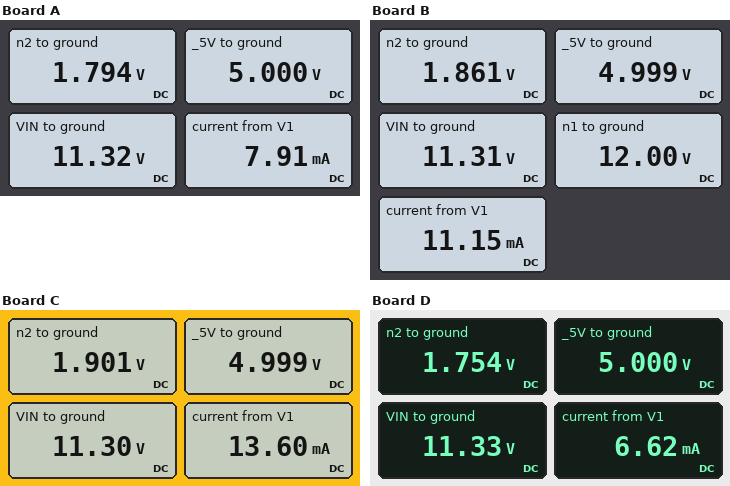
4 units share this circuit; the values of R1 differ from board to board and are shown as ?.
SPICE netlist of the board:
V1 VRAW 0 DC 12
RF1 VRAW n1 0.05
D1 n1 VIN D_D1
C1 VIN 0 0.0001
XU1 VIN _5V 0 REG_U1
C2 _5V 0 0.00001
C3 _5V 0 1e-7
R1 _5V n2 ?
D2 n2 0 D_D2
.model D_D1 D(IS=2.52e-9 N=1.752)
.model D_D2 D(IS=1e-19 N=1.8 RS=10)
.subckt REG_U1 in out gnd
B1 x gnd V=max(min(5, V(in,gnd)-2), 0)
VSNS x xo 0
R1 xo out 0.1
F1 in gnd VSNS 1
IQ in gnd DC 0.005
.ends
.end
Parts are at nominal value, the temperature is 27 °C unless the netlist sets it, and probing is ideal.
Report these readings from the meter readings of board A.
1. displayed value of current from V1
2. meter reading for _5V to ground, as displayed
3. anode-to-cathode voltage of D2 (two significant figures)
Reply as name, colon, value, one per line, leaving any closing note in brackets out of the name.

displayed value of current from V1: 7.91 mA
meter reading for _5V to ground, as displayed: 5.000 V
anode-to-cathode voltage of D2: 1.8 V
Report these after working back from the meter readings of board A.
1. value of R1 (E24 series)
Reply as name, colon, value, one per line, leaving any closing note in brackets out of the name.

value of R1: 1.1 kΩ
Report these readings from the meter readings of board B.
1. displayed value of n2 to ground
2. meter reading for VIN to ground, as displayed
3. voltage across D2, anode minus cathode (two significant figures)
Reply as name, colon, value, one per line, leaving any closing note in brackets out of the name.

displayed value of n2 to ground: 1.861 V
meter reading for VIN to ground, as displayed: 11.31 V
voltage across D2, anode minus cathode: 1.9 V
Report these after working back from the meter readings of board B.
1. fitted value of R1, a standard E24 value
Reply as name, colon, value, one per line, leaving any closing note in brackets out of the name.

fitted value of R1, a standard E24 value: 510 Ω
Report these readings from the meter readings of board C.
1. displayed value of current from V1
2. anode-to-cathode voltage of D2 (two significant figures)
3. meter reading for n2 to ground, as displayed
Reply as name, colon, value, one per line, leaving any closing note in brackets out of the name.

displayed value of current from V1: 13.60 mA
anode-to-cathode voltage of D2: 1.9 V
meter reading for n2 to ground, as displayed: 1.901 V
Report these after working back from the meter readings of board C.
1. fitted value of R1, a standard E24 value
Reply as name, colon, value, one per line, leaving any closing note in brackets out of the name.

fitted value of R1, a standard E24 value: 360 Ω
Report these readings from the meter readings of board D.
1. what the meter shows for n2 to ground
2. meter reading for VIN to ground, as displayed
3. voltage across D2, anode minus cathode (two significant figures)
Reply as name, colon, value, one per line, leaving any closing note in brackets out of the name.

what the meter shows for n2 to ground: 1.754 V
meter reading for VIN to ground, as displayed: 11.33 V
voltage across D2, anode minus cathode: 1.8 V
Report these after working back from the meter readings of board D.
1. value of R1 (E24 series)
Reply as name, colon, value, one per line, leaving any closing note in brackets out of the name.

value of R1: 2 kΩ
